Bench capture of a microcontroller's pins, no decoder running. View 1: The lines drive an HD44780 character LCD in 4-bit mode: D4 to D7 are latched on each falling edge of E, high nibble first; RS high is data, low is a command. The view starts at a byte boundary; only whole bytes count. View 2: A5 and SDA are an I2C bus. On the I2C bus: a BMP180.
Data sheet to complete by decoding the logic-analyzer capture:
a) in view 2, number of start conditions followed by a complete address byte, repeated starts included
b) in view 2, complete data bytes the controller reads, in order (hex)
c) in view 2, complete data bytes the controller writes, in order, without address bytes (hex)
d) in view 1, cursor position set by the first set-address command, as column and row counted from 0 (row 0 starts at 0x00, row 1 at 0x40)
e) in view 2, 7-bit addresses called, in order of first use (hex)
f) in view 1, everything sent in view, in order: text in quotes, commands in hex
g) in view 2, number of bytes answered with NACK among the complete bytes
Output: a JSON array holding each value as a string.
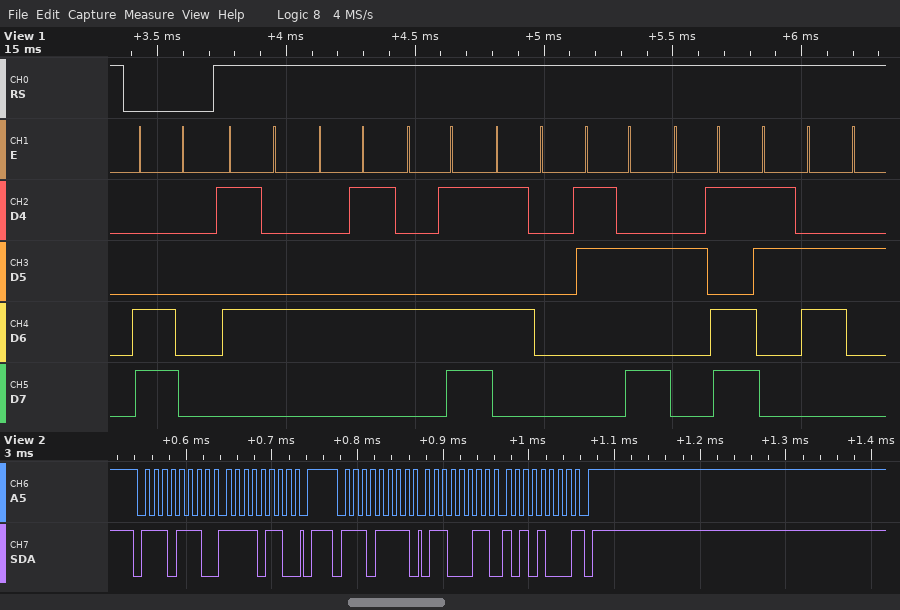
["2", "63 A8", "F6", "column 0, row 1", "0x77", "0xC0 \"TEMP:-6\"", "1"]
